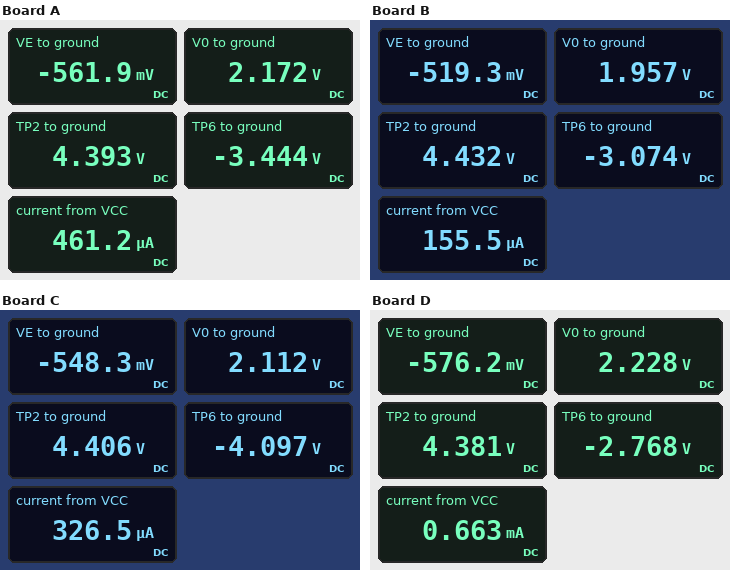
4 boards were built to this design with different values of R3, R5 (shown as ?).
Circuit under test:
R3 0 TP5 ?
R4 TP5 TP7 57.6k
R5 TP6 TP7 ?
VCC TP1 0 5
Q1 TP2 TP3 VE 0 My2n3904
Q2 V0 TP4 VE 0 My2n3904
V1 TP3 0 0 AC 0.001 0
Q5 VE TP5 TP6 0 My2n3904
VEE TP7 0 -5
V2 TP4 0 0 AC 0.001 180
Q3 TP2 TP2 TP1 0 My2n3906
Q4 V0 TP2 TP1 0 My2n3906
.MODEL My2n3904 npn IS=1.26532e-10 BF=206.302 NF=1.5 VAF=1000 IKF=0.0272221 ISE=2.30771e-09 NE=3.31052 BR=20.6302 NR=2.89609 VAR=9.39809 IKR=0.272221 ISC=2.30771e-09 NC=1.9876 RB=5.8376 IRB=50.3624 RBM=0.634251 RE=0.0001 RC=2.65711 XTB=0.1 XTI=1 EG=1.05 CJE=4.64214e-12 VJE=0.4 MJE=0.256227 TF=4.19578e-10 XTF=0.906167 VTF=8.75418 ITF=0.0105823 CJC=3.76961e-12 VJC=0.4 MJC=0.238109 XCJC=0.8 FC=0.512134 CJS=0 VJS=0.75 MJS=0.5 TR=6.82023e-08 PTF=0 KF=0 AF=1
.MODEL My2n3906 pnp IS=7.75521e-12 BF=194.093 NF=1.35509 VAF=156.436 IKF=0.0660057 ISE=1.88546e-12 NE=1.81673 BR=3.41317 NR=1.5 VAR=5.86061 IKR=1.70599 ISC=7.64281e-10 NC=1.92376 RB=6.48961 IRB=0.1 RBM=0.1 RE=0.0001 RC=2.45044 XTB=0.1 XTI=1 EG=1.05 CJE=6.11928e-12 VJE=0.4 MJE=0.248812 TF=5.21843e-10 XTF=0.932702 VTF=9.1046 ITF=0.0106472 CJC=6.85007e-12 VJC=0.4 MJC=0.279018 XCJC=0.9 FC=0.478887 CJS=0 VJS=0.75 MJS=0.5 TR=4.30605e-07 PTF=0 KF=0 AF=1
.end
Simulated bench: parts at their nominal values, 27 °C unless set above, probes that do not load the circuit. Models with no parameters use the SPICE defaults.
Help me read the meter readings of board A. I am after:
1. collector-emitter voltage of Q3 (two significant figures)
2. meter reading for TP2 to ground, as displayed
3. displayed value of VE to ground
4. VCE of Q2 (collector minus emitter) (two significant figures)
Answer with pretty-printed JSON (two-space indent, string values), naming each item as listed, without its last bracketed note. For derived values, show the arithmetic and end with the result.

{
  "collector-emitter voltage of Q3": "4.393 V - 5 V = -610 mV",
  "meter reading for TP2 to ground, as displayed": "4.393 V",
  "displayed value of VE to ground": "-561.9 mV",
  "VCE of Q2 (collector minus emitter)": "2.172 V - (-561.9 mV) = 2.7 V"
}
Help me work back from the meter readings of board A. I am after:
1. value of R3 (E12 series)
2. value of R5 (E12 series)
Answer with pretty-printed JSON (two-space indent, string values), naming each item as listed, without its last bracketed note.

{
  "value of R3": "68 kΩ",
  "value of R5": "3.3 kΩ"
}
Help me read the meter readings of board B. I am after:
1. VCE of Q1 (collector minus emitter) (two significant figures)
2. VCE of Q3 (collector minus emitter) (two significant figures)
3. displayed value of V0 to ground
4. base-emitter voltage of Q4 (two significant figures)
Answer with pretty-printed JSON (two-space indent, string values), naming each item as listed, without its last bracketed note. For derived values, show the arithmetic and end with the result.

{
  "VCE of Q1 (collector minus emitter)": "4.432 V - (-519.3 mV) = 5.0 V",
  "VCE of Q3 (collector minus emitter)": "4.432 V - 5 V = -570 mV",
  "displayed value of V0 to ground": "1.957 V",
  "base-emitter voltage of Q4": "4.432 V - 5 V = -570 mV"
}
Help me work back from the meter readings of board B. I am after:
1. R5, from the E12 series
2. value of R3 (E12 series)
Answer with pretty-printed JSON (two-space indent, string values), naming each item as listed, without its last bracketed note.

{
  "R5, from the E12 series": "12 kΩ",
  "value of R3": "56 kΩ"
}
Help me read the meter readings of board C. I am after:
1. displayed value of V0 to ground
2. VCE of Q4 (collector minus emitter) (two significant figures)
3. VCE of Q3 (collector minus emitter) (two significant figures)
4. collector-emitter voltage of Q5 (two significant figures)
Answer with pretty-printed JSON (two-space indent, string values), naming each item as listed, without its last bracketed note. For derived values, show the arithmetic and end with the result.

{
  "displayed value of V0 to ground": "2.112 V",
  "VCE of Q4 (collector minus emitter)": "2.112 V - 5 V = -2.9 V",
  "VCE of Q3 (collector minus emitter)": "4.406 V - 5 V = -590 mV",
  "collector-emitter voltage of Q5": "-548.3 mV - (-4.097 V) = 3.5 V"
}
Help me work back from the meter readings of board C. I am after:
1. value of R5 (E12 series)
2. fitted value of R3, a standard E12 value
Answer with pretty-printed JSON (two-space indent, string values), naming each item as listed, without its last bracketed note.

{
  "value of R5": "2.7 kΩ",
  "fitted value of R3, a standard E12 value": "120 kΩ"
}
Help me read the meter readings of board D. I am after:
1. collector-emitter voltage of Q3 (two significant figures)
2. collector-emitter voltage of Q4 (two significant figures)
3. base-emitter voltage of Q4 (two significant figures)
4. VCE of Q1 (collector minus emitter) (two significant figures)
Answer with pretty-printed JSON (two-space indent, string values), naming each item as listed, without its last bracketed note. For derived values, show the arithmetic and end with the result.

{
  "collector-emitter voltage of Q3": "4.381 V - 5 V = -620 mV",
  "collector-emitter voltage of Q4": "2.228 V - 5 V = -2.8 V",
  "base-emitter voltage of Q4": "4.381 V - 5 V = -620 mV",
  "VCE of Q1 (collector minus emitter)": "4.381 V - (-576.2 mV) = 5.0 V"
}
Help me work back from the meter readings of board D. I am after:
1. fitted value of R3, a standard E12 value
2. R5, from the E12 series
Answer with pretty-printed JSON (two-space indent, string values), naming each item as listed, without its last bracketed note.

{
  "fitted value of R3, a standard E12 value": "39 kΩ",
  "R5, from the E12 series": "3.3 kΩ"
}
